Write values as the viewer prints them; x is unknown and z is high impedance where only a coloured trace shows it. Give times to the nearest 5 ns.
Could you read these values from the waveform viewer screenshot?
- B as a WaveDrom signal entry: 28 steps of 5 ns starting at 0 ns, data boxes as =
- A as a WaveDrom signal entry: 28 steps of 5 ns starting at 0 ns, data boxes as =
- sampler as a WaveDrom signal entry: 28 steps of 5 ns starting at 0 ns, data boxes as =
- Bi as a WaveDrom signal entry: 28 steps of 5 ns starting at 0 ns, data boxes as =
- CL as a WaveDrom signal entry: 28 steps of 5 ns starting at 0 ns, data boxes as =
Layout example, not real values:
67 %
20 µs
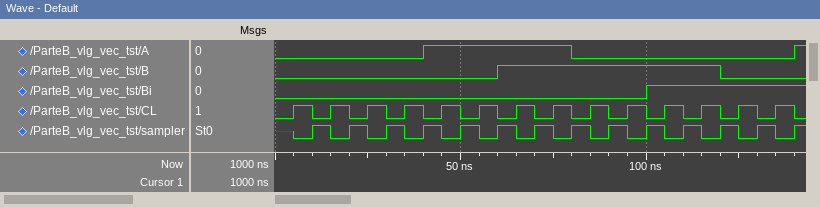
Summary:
{name: 'B', wave: '0...........1...........0...'}
{name: 'A', wave: '0.......1.......0...........'}
{name: 'sampler', wave: 'x010101010101010101010101010'}
{name: 'Bi', wave: '0...................1.......'}
{name: 'CL', wave: '0101010101010101010101010101'}
